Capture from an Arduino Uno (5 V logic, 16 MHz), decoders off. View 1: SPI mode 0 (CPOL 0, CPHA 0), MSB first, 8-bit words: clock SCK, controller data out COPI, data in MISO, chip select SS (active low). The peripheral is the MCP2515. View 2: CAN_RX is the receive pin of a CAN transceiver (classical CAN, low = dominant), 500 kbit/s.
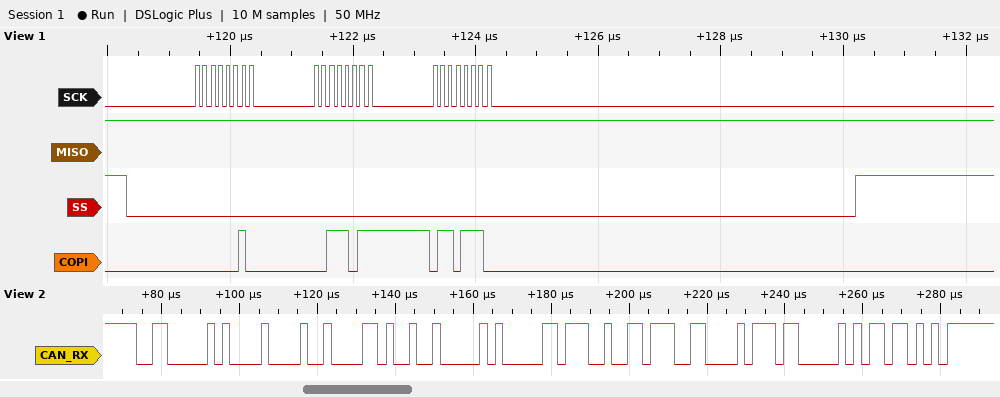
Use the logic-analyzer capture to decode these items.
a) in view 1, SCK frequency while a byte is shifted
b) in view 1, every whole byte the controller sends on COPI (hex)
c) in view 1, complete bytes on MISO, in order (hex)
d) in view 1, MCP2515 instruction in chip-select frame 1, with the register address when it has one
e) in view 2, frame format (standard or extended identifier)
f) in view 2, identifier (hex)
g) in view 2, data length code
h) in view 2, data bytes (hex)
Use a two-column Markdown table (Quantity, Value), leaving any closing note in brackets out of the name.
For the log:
| Quantity | Value |
|---|---|
| in view 1, SCK frequency while a byte is shifted | 8 MHz |
| in view 1, every whole byte the controller sends on COPI | 02 3B 6E |
| in view 1, complete bytes on MISO, in order | FF FF FF |
| in view 1, MCP2515 instruction in chip-select frame 1, with the register address when it has one | WRITE 0x3B |
| in view 2, frame format | standard |
| in view 2, identifier | 0x302 |
| in view 2, data length code | 8 |
| in view 2, data bytes | 48 69 20 41 72 6E 61 76 |
